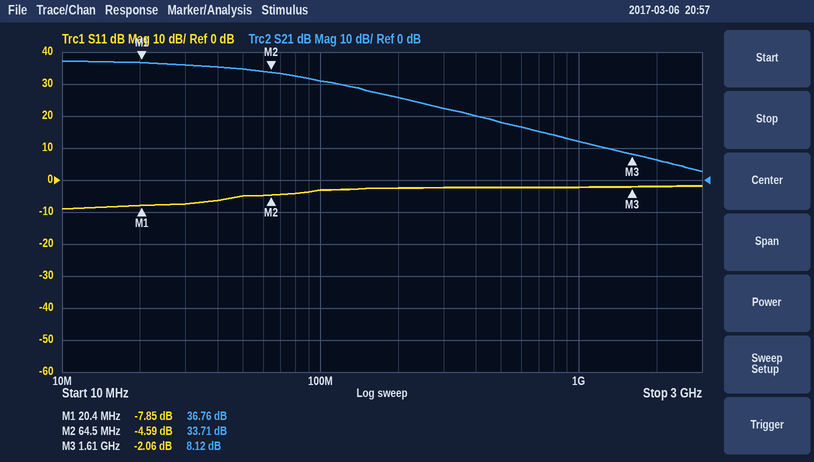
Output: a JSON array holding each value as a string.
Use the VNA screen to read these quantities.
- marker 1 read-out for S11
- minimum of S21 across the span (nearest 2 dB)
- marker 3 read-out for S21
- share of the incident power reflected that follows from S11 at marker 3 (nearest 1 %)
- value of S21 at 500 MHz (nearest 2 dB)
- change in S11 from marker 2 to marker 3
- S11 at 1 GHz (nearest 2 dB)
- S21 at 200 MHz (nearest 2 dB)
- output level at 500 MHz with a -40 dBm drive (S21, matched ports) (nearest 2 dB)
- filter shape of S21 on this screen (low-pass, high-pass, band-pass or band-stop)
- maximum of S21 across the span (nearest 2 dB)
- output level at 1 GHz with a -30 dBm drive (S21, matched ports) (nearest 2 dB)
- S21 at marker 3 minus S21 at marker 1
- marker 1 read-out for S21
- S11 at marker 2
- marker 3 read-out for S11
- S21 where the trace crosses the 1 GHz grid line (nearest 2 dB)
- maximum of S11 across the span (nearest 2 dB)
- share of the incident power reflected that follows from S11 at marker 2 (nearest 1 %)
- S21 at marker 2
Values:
["-7.85 dB", "2 dB", "8.12 dB", "62 %", "18 dB", "2.53 dB", "-2 dB", "26 dB", "-22 dBm", "low-pass", "38 dB", "-18 dBm", "-28.64 dB", "36.76 dB", "-4.59 dB", "-2.06 dB", "12 dB", "-2 dB", "35 %", "33.71 dB"]
